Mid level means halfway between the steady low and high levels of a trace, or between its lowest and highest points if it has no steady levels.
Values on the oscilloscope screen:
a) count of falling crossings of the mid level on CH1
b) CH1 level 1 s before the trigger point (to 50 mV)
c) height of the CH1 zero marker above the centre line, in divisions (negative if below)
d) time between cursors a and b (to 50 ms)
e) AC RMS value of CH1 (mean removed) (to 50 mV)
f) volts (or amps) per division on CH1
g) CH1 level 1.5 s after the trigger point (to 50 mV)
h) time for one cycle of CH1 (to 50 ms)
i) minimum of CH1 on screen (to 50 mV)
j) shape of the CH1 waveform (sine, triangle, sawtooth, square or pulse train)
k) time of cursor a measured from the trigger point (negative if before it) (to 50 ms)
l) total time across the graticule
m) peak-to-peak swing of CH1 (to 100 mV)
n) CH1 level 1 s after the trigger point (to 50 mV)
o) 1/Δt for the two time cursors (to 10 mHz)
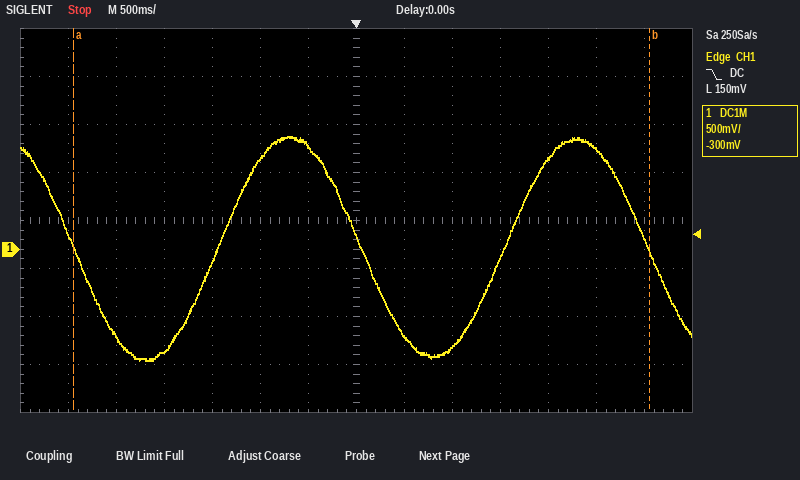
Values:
3
950 mV
-0.6 div
6.00 s
800 mV
500 mV
-100 mV
3.00 s
-1.15 V
sine
-2.95 s
7 s
2.30 V
-1.00 V
170 mHz
